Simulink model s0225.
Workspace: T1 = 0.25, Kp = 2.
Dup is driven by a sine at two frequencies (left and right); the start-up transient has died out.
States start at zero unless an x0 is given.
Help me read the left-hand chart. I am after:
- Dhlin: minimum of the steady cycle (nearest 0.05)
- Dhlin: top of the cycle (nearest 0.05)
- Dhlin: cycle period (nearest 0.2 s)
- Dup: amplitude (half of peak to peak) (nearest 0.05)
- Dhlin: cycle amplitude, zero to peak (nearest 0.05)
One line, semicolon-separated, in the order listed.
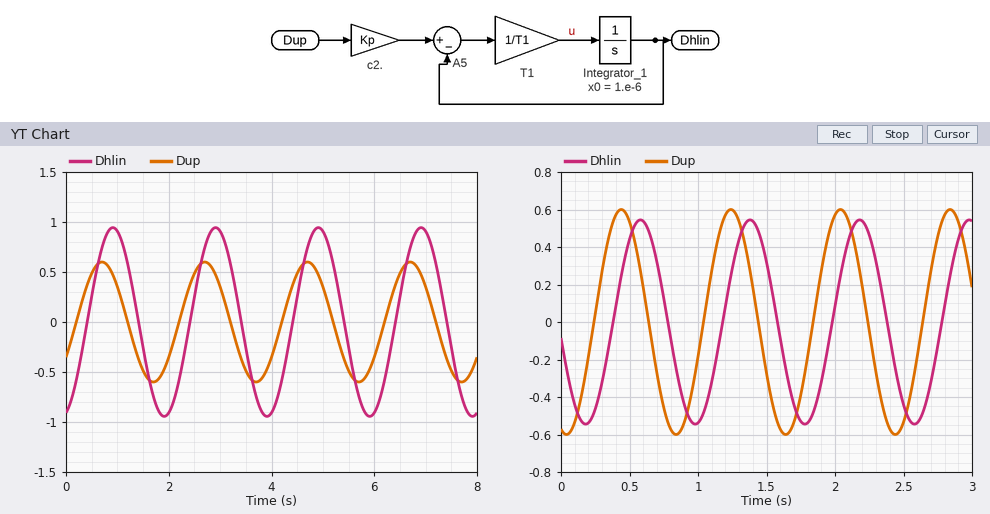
-0.95; 0.95; 2.0 s; 0.60; 0.95
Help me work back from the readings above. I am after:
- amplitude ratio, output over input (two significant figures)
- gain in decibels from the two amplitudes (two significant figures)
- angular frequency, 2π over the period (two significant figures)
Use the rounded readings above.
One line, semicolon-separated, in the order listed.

1.6; 4.0 dB; 3.1 rad/s
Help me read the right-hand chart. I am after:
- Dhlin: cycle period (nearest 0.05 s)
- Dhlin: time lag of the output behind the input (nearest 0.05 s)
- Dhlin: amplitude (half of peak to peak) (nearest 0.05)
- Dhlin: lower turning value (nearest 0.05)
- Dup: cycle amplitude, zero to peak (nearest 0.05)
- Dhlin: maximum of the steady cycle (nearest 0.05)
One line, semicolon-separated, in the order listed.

0.80 s; 0.15 s; 0.55; -0.55; 0.60; 0.55
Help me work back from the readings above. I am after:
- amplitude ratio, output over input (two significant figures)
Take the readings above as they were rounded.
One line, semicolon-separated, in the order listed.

0.92
